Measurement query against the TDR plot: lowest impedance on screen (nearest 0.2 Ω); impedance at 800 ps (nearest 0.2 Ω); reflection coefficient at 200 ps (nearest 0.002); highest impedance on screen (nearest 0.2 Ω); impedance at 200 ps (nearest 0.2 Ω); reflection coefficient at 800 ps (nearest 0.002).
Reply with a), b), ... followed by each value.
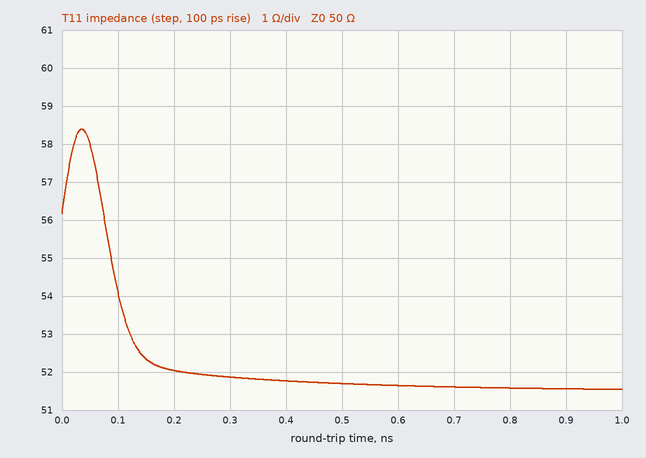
a) 51.6 Ω
b) 51.6 Ω
c) +0.020
d) 58.4 Ω
e) 52.0 Ω
f) +0.016
